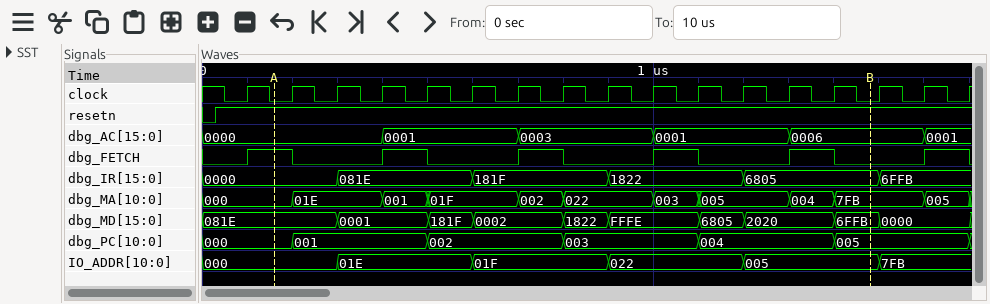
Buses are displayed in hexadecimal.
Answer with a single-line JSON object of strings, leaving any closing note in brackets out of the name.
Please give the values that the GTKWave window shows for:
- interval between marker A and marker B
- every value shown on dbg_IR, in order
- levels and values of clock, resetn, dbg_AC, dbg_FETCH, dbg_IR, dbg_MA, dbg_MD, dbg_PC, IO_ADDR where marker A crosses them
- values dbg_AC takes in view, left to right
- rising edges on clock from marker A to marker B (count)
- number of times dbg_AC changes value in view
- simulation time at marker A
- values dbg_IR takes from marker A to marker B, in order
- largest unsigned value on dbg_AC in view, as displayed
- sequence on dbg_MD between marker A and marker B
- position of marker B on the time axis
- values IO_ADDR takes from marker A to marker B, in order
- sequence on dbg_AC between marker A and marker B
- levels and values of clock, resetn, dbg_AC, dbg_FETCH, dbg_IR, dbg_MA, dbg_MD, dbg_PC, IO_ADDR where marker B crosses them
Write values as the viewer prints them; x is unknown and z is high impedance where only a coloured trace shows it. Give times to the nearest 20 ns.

{"interval between marker A and marker B": "1320 ns", "every value shown on dbg_IR, in order": "0000, 081E, 181F, 1822, 6805, 6FFB", "levels and values of clock, resetn, dbg_AC, dbg_FETCH, dbg_IR, dbg_MA, dbg_MD, dbg_PC, IO_ADDR where marker A crosses them": "clock=0, resetn=1, dbg_AC=0000, dbg_FETCH=1, dbg_IR=0000, dbg_MA=000, dbg_MD=081E, dbg_PC=000, IO_ADDR=000", "values dbg_AC takes in view, left to right": "0000, 0001, 0003, 0001, 0006, 0001", "rising edges on clock from marker A to marker B": "13", "number of times dbg_AC changes value in view": "5", "simulation time at marker A": "160 ns", "values dbg_IR takes from marker A to marker B, in order": "0000, 081E, 181F, 1822, 6805", "largest unsigned value on dbg_AC in view, as displayed": "0006", "sequence on dbg_MD between marker A and marker B": "081E, 0001, 181F, 0002, 1822, FFFE, 6805, 2020, 6FFB", "position of marker B on the time axis": "1480 ns", "values IO_ADDR takes from marker A to marker B, in order": "000, 01E, 01F, 022, 005", "sequence on dbg_AC between marker A and marker B": "0000, 0001, 0003, 0001, 0006", "levels and values of clock, resetn, dbg_AC, dbg_FETCH, dbg_IR, dbg_MA, dbg_MD, dbg_PC, IO_ADDR where marker B crosses them": "clock=0, resetn=1, dbg_AC=0006, dbg_FETCH=0, dbg_IR=6805, dbg_MA=7FB, dbg_MD=6FFB, dbg_PC=005, IO_ADDR=005"}
